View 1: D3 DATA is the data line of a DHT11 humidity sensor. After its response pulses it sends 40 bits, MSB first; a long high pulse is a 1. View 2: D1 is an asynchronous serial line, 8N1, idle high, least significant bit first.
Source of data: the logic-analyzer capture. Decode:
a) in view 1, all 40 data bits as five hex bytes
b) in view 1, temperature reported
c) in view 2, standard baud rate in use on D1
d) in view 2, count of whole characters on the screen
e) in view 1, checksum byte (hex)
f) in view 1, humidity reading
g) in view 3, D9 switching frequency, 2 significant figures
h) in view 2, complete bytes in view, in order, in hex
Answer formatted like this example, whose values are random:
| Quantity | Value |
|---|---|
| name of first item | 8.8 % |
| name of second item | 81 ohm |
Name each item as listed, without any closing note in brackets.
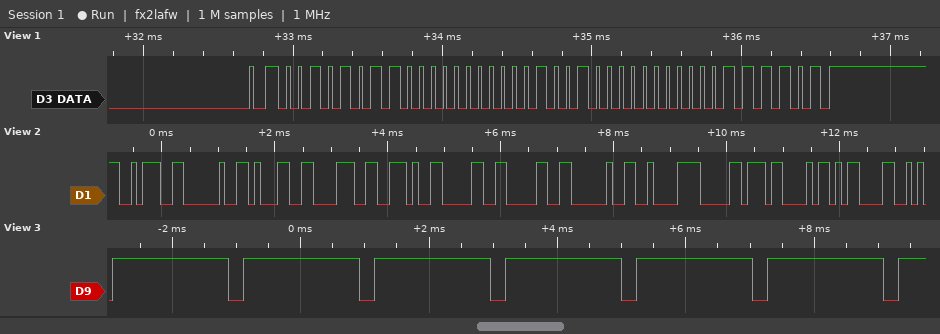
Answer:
| Quantity | Value |
|---|---|
| in view 1, all 40 data bits as five hex bytes | 2B 00 12 00 3D |
| in view 1, temperature reported | 18.0 °C |
| in view 2, standard baud rate in use on D1 | 9600 baud |
| in view 2, count of whole characters on the screen | 12 |
| in view 1, checksum byte | 0x3D |
| in view 1, humidity reading | 43 % |
| in view 3, D9 switching frequency, 2 significant figures | 490 Hz |
| in view 2, complete bytes in view, in order, in hex | 3A 20 31 38 2E 30 30 20 C2 B0 43 0D |
